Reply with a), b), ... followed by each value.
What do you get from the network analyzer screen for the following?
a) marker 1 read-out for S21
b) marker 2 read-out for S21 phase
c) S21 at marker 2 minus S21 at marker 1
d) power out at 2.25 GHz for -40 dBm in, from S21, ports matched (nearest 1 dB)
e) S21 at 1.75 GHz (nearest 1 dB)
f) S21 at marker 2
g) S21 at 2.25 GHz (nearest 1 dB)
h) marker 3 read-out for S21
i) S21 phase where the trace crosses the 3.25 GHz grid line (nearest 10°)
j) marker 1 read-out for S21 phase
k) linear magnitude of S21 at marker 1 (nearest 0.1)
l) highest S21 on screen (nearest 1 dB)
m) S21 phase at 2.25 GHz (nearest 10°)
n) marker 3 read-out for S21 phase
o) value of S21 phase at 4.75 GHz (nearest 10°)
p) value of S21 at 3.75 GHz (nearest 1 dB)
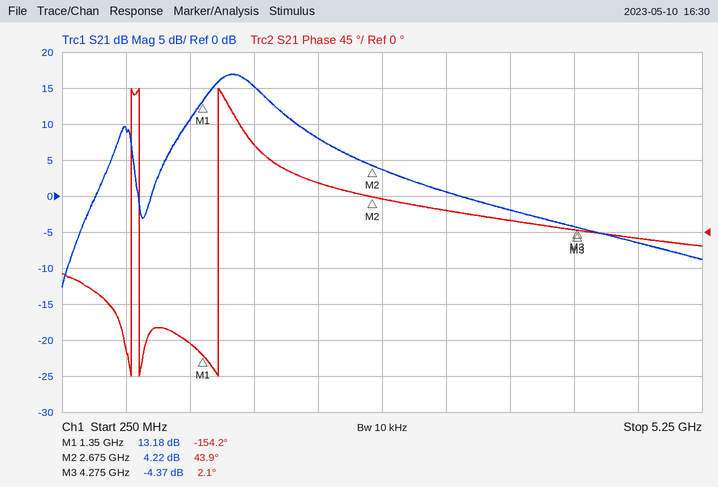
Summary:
a) 13.18 dB
b) 43.9°
c) -8.96 dB
d) -32 dBm
e) 15 dB
f) 4.22 dB
g) 8 dB
h) -4.37 dB
i) 30°
j) -154.2°
k) 4.6
l) 17 dB
m) 60°
n) 2.1°
o) -10°
p) -2 dB
